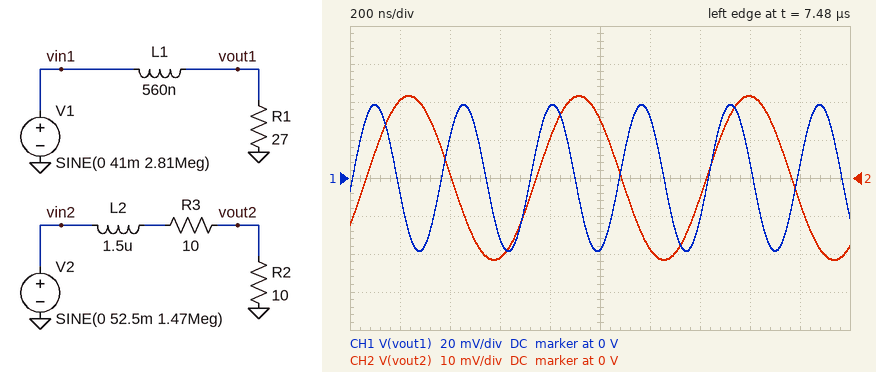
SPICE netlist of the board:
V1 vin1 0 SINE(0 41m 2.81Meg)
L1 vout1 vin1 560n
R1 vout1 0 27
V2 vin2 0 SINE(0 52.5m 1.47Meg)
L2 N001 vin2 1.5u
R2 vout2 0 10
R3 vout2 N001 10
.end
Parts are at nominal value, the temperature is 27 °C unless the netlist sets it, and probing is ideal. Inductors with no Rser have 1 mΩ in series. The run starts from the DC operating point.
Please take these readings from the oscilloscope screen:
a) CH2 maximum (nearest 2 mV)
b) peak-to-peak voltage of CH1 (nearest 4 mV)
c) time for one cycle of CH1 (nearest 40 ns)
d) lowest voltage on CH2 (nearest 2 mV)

22 mV
76 mV
360 ns
-22 mV
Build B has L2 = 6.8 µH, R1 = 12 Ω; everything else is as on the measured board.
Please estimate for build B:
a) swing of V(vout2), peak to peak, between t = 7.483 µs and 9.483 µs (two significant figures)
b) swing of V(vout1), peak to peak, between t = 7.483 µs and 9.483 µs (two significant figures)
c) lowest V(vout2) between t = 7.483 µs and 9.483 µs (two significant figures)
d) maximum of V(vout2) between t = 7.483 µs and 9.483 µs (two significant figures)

16 mV
63 mV
-8.0 mV
8.0 mV
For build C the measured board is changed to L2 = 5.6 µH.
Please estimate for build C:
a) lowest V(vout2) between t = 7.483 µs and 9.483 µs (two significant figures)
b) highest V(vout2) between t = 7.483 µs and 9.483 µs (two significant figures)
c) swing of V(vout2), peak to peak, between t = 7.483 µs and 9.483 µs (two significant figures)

-9.5 mV
9.5 mV
19 mV
